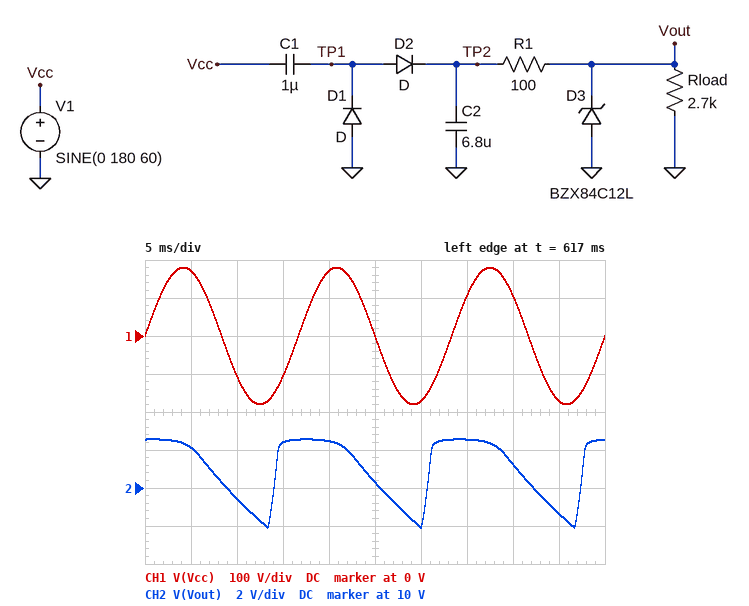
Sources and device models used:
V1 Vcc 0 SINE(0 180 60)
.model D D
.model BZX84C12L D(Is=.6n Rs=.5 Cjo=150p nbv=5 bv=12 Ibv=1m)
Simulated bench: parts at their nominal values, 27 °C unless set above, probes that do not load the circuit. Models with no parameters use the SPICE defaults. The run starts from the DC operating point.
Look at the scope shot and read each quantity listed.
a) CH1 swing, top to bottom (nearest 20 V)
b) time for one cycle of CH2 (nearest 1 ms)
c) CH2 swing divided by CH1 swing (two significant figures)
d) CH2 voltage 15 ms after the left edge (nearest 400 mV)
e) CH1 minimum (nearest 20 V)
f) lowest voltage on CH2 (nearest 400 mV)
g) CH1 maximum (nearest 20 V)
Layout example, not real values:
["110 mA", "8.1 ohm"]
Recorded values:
["360 V", "17 ms", "0.013", "12.4 V", "-180 V", "8.0 V", "180 V"]
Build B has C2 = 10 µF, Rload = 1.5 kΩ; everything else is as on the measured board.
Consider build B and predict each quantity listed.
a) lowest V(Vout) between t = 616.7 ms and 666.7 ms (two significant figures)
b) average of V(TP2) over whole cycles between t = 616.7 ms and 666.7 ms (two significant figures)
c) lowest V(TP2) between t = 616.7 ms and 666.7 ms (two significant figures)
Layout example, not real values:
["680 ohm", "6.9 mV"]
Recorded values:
["7.4 V", "13 V", "7.9 V"]
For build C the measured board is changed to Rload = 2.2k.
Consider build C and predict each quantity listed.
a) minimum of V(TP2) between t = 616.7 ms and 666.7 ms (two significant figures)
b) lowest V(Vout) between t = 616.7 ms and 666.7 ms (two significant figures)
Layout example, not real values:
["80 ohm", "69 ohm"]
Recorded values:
["7.5 V", "7.2 V"]
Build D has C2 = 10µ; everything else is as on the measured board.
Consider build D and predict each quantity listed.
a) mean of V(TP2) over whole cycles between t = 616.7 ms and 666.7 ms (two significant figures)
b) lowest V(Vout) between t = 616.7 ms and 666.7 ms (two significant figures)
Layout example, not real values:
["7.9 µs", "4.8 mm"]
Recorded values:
["14 V", "9.3 V"]
